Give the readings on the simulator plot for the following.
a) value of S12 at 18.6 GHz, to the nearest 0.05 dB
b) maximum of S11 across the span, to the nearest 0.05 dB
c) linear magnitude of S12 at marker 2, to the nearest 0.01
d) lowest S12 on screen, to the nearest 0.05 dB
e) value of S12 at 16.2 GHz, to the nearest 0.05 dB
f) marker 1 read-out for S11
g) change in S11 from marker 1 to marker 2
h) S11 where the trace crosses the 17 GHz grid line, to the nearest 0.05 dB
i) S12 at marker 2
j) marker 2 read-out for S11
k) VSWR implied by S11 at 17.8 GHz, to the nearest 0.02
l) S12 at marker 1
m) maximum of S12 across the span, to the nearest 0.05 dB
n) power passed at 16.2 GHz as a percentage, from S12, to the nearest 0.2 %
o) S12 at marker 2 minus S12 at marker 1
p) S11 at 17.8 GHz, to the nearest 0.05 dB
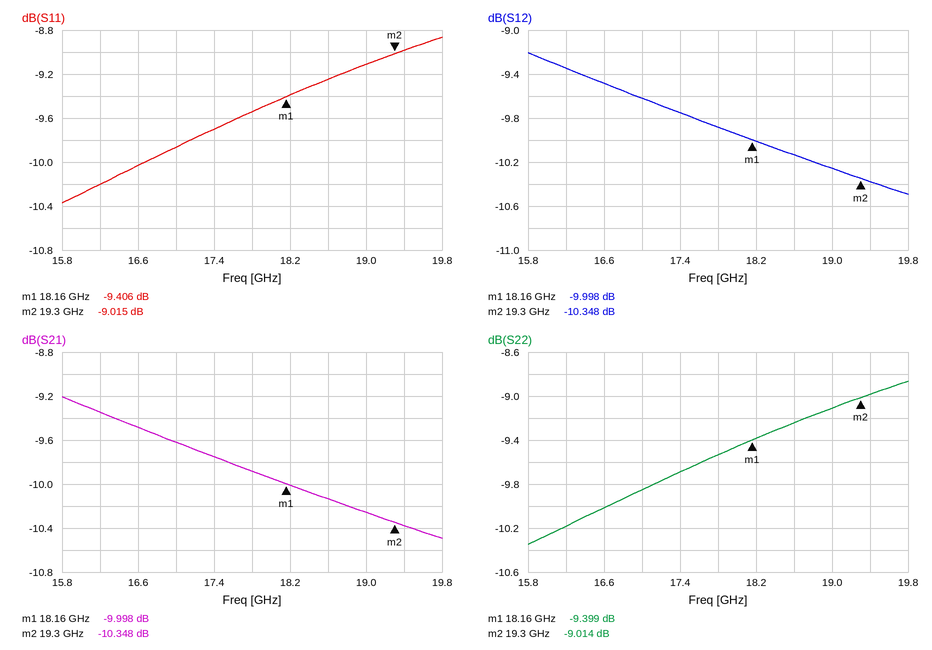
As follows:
-10.15 dB
-8.85 dB
0.30
-10.50 dB
-9.35 dB
-9.406 dB
0.391 dB
-9.85 dB
-10.348 dB
-9.015 dB
2.00
-9.998 dB
-9.20 dB
11.6 %
-0.350 dB
-9.55 dB
